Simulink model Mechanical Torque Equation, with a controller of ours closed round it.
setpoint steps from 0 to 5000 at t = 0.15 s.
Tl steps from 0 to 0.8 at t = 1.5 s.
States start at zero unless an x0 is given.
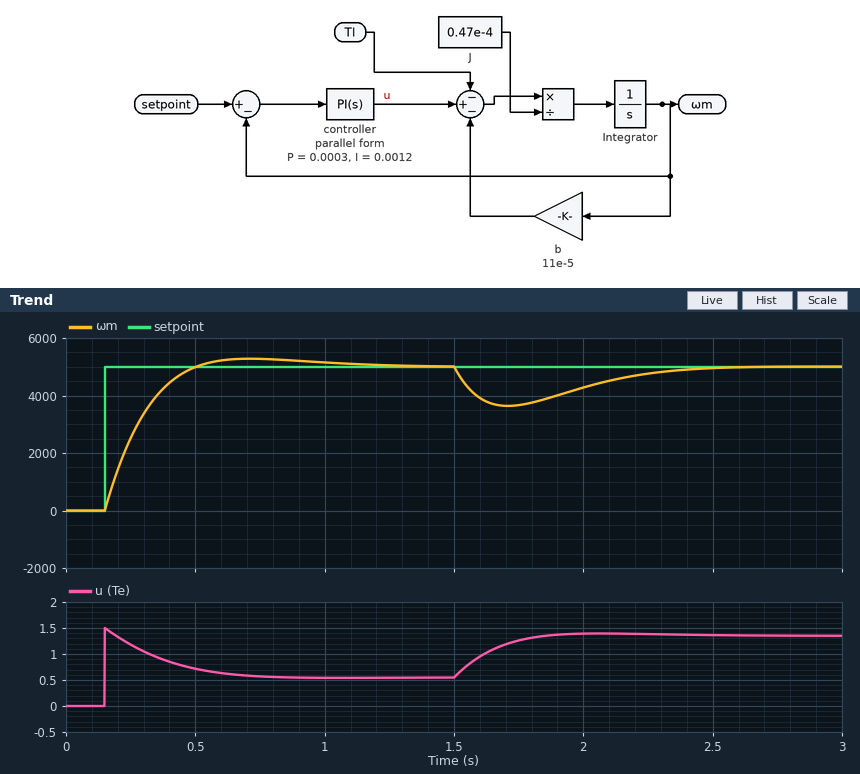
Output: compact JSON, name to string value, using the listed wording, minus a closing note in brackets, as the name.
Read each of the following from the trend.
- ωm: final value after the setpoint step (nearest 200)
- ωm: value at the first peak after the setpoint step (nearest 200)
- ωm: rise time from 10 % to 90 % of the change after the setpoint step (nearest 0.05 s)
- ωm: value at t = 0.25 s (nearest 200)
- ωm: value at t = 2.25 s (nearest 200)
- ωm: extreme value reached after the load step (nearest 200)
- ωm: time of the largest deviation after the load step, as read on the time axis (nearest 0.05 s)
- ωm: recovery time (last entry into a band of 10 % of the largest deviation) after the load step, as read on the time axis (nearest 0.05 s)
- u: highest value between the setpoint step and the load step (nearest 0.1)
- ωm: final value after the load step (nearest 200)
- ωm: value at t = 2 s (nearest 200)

{"ωm: final value after the setpoint step": "5000", "ωm: value at the first peak after the setpoint step": "5200", "ωm: rise time from 10 % to 90 % of the change after the setpoint step": "0.25 s", "ωm: value at t = 0.25 s": "2600", "ωm: value at t = 2.25 s": "4800", "ωm: extreme value reached after the load step": "3600", "ωm: time of the largest deviation after the load step, as read on the time axis": "1.70 s", "ωm: recovery time (last entry into a band of 10 % of the largest deviation) after the load step, as read on the time axis": "2.35 s", "u: highest value between the setpoint step and the load step": "1.5", "ωm: final value after the load step": "5000", "ωm: value at t = 2 s": "4200"}
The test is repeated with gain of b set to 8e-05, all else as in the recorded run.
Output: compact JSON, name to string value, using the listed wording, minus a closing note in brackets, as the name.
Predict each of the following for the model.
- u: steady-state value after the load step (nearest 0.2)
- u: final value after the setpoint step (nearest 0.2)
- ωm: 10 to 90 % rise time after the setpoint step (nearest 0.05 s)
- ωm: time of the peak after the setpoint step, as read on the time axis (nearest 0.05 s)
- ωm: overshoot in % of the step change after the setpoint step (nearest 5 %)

{"u: steady-state value after the load step": "1.2", "u: final value after the setpoint step": "0.4", "ωm: 10 to 90 % rise time after the setpoint step": "0.20 s", "ωm: time of the peak after the setpoint step, as read on the time axis": "0.65 s", "ωm: overshoot in % of the step change after the setpoint step": "10 %"}
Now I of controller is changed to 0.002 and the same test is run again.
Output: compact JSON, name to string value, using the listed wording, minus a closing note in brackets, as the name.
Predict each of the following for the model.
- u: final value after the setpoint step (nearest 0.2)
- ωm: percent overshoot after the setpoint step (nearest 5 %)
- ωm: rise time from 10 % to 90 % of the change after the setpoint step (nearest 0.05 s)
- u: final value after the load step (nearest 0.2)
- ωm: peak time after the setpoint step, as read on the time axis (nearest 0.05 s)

{"u: final value after the setpoint step": "0.6", "ωm: percent overshoot after the setpoint step": "15 %", "ωm: rise time from 10 % to 90 % of the change after the setpoint step": "0.20 s", "u: final value after the load step": "1.4", "ωm: peak time after the setpoint step, as read on the time axis": "0.55 s"}
